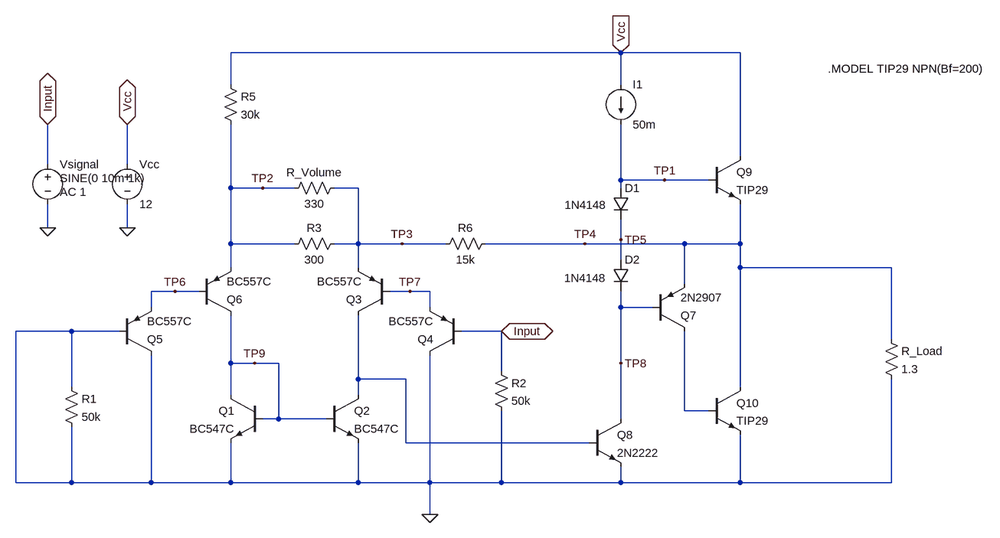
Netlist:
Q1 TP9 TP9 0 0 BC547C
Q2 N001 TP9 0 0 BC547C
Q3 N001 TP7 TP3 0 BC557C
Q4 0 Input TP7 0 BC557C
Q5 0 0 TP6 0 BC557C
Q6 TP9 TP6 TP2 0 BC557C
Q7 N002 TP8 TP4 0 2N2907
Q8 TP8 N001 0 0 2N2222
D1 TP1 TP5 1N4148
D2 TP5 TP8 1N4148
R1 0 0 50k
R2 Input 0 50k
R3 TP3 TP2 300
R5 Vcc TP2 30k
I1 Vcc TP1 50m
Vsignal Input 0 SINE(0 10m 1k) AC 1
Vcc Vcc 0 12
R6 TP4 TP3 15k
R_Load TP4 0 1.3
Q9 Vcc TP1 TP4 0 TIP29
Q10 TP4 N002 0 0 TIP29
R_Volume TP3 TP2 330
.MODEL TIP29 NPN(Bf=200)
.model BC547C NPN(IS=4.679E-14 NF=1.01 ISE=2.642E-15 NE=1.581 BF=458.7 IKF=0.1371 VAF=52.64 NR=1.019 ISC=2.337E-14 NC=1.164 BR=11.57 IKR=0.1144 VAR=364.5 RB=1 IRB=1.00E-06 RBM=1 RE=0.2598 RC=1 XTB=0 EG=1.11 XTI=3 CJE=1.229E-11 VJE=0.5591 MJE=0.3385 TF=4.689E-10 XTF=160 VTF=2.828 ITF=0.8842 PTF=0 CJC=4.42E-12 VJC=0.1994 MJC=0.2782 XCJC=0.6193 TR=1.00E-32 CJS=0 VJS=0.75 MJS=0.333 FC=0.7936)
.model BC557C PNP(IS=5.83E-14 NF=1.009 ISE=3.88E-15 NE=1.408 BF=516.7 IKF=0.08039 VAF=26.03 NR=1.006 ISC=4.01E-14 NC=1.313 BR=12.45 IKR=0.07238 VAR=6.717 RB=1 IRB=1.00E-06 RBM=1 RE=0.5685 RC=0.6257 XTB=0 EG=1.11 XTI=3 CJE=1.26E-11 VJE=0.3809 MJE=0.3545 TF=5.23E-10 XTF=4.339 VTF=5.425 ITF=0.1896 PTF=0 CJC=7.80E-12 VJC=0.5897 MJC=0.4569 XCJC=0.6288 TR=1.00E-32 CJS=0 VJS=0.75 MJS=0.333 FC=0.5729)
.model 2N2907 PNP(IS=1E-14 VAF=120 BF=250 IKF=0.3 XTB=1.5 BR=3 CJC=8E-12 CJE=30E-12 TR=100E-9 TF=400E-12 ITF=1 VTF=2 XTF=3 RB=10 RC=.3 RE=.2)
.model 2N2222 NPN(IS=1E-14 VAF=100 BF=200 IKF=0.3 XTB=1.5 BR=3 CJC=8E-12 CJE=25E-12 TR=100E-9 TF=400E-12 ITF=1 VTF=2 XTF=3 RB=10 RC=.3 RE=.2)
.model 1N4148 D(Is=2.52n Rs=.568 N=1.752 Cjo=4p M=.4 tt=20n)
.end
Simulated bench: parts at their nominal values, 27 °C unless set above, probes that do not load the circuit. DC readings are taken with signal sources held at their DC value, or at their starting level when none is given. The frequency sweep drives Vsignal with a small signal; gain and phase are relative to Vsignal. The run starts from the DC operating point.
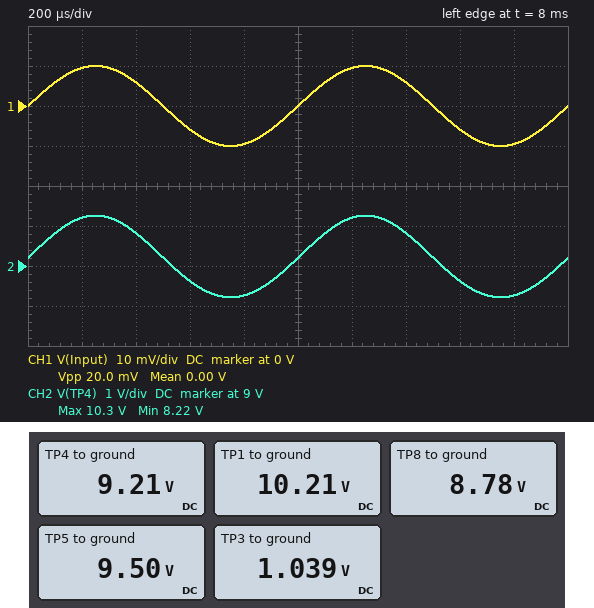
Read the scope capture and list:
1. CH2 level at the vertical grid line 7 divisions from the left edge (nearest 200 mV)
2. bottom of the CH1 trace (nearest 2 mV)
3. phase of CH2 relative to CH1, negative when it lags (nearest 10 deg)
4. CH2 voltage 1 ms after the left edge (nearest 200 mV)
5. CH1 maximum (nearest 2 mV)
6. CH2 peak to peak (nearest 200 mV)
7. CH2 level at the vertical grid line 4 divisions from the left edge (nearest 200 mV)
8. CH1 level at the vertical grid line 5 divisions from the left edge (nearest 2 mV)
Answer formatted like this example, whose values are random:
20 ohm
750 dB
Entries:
9.8 V
-10 mV
0 deg
9.2 V
10 mV
2.0 V
8.2 V
0 V
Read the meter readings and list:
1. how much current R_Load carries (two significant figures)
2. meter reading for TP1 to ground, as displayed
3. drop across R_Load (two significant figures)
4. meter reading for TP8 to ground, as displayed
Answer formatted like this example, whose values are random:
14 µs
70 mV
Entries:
7.1 A
10.21 V
9.2 V
8.78 V
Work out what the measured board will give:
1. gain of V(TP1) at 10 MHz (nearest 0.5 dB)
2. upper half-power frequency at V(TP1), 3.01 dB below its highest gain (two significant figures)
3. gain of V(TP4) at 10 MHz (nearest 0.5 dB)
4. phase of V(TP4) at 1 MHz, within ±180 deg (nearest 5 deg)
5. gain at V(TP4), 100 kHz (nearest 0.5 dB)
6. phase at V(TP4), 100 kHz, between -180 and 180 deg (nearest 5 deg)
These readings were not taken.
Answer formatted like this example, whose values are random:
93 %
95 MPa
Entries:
19.0 dB
190 kHz
19.0 dB
-40 deg
39.0 dB
-20 deg
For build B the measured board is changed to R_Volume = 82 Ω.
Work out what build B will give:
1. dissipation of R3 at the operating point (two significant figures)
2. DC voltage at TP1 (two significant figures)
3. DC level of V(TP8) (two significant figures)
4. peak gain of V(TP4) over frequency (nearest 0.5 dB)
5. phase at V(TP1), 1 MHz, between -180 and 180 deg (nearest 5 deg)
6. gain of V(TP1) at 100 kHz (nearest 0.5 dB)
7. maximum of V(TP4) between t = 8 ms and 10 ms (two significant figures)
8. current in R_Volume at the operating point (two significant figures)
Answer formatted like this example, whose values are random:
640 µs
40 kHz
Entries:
120 nW
11 V
9.7 V
45.5 dB
-40 deg
43.5 dB
12 V
73 µA
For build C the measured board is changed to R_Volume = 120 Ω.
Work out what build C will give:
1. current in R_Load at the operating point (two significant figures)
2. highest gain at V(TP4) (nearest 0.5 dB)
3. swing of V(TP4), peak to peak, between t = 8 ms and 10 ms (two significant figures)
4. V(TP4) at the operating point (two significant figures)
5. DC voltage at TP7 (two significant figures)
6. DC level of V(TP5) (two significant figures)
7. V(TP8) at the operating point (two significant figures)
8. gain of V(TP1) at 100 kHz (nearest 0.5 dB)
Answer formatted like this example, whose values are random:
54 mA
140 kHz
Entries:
7.5 A
44.0 dB
3.1 V
9.8 V
440 mV
10 V
9.4 V
42.0 dB
